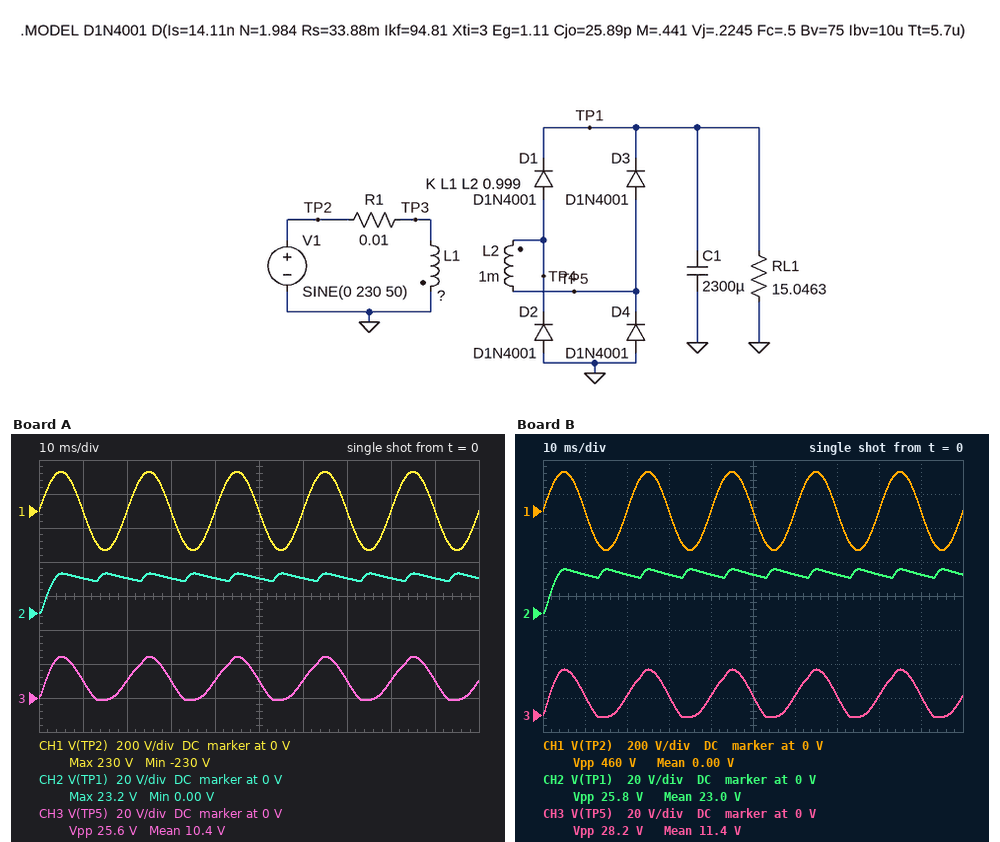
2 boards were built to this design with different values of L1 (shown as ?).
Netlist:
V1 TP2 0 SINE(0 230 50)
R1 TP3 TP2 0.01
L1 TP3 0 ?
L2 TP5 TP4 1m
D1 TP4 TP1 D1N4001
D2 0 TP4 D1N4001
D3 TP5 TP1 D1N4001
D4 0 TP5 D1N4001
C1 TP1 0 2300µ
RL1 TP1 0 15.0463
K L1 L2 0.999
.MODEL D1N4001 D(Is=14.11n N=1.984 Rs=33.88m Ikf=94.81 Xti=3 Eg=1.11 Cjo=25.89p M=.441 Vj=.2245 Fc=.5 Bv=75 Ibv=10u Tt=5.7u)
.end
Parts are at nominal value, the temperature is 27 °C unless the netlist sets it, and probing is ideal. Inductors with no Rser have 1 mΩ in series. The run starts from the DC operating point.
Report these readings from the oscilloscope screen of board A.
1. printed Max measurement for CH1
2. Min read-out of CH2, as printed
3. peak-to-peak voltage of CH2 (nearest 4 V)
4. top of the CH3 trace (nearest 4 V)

230 V
0.00 V
24 V
24 V
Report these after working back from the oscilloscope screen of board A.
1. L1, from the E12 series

82 mH
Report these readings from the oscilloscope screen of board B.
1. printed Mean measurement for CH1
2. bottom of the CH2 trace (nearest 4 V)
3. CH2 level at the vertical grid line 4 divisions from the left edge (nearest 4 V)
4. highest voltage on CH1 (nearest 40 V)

0.00 V
0 V
24 V
240 V
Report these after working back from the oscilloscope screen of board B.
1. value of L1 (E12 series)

68 mH
